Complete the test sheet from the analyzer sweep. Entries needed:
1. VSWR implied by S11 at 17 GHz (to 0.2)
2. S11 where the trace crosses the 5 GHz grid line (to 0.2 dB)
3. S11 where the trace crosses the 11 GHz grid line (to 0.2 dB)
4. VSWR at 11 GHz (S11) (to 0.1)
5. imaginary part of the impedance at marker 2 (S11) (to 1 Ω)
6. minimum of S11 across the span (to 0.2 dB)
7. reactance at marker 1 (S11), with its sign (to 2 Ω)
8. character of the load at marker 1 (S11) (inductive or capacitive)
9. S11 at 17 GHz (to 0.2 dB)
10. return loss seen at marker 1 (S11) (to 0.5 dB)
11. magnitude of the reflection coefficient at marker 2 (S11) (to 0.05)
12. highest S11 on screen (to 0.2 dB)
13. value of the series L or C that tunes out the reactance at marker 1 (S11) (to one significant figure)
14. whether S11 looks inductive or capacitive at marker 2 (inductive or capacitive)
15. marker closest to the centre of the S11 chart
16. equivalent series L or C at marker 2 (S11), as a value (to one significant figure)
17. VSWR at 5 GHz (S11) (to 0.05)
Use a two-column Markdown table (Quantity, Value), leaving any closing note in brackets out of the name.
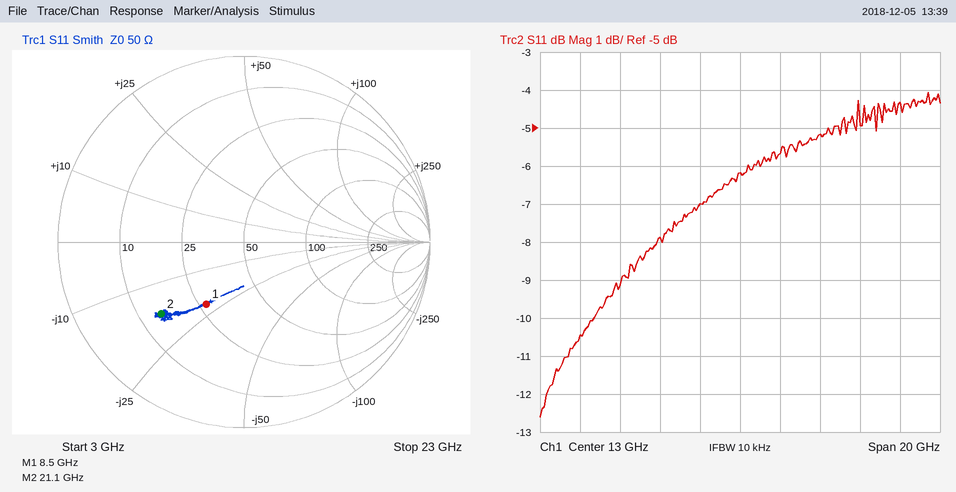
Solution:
| Quantity | Value |
|---|---|
| VSWR implied by S11 at 17 GHz | 3.4 |
| S11 where the trace crosses the 5 GHz grid line | -10.4 dB |
| S11 where the trace crosses the 11 GHz grid line | -7.0 dB |
| VSWR at 11 GHz (S11) | 2.6 |
| imaginary part of the impedance at marker 2 (S11) | -17 Ω |
| minimum of S11 across the span | -12.6 dB |
| reactance at marker 1 (S11), with its sign | -22 Ω |
| character of the load at marker 1 (S11) | capacitive |
| S11 at 17 GHz | -5.2 dB |
| return loss seen at marker 1 (S11) | 8.0 dB |
| magnitude of the reflection coefficient at marker 2 (S11) | 0.60 |
| highest S11 on screen | -4.0 dB |
| value of the series L or C that tunes out the reactance at marker 1 (S11) | 400 pH |
| whether S11 looks inductive or capacitive at marker 2 | capacitive |
| marker closest to the centre of the S11 chart | marker 1 |
| equivalent series L or C at marker 2 (S11), as a value | 400 fF |
| VSWR at 5 GHz (S11) | 1.85 |
